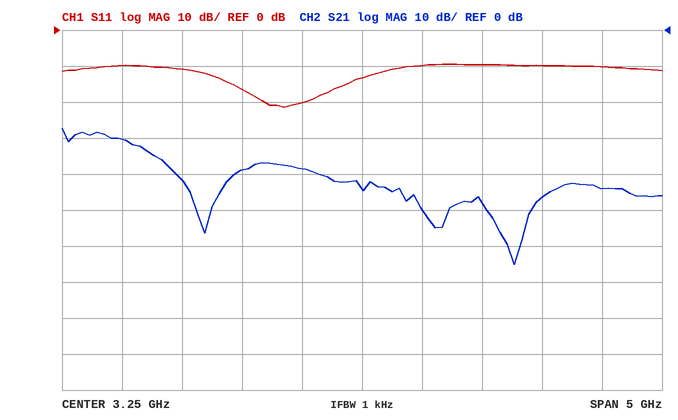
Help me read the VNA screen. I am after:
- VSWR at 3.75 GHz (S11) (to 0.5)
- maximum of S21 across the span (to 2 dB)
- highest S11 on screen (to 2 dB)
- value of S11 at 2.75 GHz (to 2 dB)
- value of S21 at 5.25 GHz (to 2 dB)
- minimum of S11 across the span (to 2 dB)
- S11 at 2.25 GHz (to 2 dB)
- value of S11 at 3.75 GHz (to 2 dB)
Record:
2.0
-28 dB
-10 dB
-20 dB
-44 dB
-22 dB
-16 dB
-10 dB
